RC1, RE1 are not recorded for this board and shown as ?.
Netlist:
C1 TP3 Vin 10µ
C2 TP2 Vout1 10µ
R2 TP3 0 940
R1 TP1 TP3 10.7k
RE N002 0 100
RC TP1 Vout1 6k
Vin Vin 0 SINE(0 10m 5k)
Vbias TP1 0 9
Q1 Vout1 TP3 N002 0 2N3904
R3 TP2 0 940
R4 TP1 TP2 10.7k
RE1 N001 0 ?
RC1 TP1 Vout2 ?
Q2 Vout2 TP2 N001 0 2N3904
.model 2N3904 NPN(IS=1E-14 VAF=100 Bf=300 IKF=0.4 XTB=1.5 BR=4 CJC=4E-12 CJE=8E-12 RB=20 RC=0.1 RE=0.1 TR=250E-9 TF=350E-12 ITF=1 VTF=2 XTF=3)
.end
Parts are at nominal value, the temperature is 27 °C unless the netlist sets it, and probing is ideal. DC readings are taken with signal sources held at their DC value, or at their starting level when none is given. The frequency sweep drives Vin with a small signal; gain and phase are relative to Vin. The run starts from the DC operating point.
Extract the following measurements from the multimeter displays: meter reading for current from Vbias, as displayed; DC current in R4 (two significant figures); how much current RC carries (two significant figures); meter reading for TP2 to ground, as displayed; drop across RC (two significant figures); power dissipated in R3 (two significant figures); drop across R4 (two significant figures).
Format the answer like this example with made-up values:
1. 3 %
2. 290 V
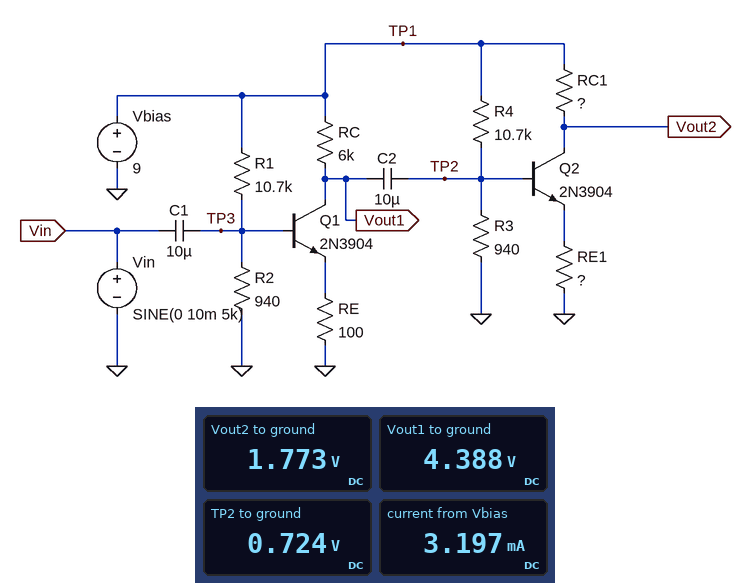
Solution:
1. 3.197 mA
2. 770 µA
3. 770 µA
4. 0.724 V
5. 4.6 V
6. 560 µW
7. 8.3 V
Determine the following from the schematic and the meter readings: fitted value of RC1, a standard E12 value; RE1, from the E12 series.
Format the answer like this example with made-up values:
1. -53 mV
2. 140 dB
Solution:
1. 8.2 kΩ
2. 82 Ω
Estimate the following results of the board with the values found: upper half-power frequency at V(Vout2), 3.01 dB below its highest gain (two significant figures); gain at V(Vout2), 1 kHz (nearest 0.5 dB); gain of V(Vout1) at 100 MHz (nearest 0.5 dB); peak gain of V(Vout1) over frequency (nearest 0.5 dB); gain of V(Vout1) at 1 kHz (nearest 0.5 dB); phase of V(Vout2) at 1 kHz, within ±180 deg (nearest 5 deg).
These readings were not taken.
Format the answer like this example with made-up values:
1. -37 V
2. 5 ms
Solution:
1. 810 kHz
2. 52.0 dB
3. -2.5 dB
4. 15.0 dB
5. 15.0 dB
6. 0 deg
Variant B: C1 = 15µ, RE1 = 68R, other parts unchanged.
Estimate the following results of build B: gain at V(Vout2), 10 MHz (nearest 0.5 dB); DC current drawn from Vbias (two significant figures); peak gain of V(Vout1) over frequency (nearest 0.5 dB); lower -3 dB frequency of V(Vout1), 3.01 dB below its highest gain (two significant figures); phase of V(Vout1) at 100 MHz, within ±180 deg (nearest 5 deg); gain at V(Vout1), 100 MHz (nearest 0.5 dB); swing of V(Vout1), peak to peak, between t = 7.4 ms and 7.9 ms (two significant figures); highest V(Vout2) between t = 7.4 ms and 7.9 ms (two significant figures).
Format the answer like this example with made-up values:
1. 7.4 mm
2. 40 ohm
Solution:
1. 28.0 dB
2. 3.3 mA
3. 17.5 dB
4. 1.9 Hz
5. 130 deg
6. -3.5 dB
7. 73 mV
8. 5.0 V
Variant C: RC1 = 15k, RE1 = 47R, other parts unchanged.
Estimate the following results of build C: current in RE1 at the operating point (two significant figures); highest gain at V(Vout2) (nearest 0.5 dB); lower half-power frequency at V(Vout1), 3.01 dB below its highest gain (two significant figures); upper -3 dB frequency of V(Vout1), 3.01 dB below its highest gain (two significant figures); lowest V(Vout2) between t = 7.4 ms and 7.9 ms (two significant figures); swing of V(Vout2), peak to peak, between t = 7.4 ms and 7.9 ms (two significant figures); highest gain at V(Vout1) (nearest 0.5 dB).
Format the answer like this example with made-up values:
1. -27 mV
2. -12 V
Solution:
1. 650 µA
2. 5.5 dB
3. 2.1 Hz
4. 25 Hz
5. 59 mV
6. 1.1 V
7. 14.5 dB
